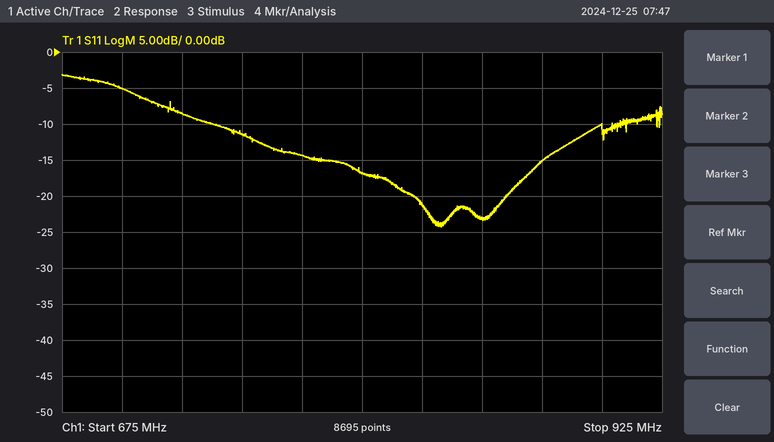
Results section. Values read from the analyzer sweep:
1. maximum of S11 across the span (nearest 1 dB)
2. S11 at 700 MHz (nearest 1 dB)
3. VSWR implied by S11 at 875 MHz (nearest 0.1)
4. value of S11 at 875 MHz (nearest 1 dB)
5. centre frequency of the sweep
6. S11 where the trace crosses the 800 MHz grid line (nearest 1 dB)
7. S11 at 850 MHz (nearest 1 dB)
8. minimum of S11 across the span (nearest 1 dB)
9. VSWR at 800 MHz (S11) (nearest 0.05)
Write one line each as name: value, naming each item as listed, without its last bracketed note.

maximum of S11 across the span: -3 dB
S11 at 700 MHz: -5 dB
VSWR implied by S11 at 875 MHz: 1.4
value of S11 at 875 MHz: -15 dB
centre frequency of the sweep: 800 MHz
S11 where the trace crosses the 800 MHz grid line: -17 dB
S11 at 850 MHz: -23 dB
minimum of S11 across the span: -24 dB
VSWR at 800 MHz (S11): 1.35
